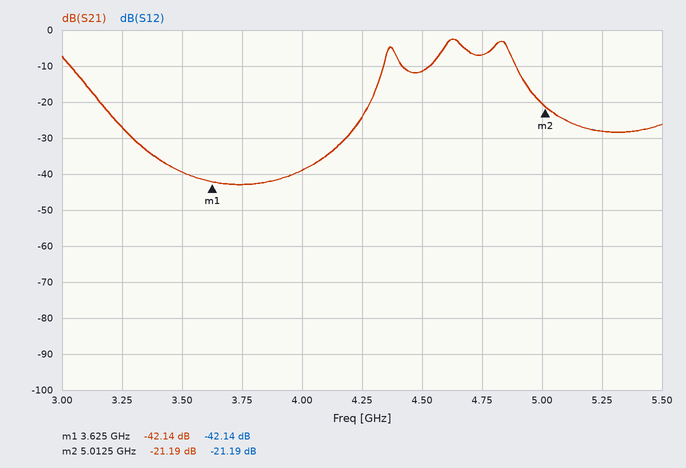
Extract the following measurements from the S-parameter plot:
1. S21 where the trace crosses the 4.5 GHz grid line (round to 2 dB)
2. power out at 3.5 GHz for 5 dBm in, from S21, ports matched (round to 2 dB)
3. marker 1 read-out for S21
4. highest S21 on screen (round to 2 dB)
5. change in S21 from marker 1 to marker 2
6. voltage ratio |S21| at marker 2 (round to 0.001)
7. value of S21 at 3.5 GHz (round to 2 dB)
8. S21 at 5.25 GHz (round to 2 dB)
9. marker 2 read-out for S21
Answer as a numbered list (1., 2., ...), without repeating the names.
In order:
1. -12 dB
2. -34 dBm
3. -42.14 dB
4. -2 dB
5. 20.95 dB
6. 0.087
7. -40 dB
8. -28 dB
9. -21.19 dB
